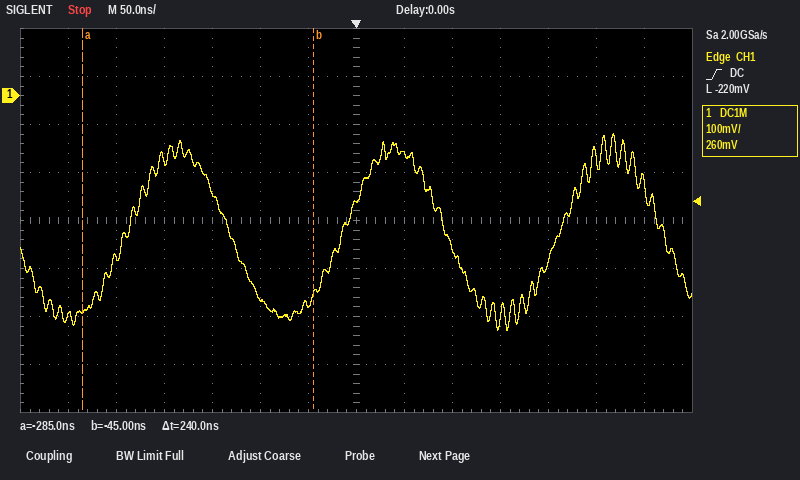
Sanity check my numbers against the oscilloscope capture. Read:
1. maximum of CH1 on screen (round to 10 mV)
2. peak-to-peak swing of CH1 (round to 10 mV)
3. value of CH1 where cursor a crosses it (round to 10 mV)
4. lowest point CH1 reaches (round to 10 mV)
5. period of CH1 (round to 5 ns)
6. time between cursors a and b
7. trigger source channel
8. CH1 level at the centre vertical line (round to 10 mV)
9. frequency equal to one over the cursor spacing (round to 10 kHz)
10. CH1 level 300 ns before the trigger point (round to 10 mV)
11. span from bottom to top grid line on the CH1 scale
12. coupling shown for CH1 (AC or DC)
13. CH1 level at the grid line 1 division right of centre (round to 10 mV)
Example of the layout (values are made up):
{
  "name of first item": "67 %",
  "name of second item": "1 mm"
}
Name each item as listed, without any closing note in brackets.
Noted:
{
  "maximum of CH1 on screen": "-80 mV",
  "peak-to-peak swing of CH1": "410 mV",
  "value of CH1 where cursor a crosses it": "-450 mV",
  "lowest point CH1 reaches": "-490 mV",
  "period of CH1": "225 ns",
  "time between cursors a and b": "240 ns",
  "trigger source channel": "CH1",
  "CH1 level at the centre vertical line": "-220 mV",
  "frequency equal to one over the cursor spacing": "4.17 MHz",
  "CH1 level 300 ns before the trigger point": "-460 mV",
  "span from bottom to top grid line on the CH1 scale": "800 mV",
  "coupling shown for CH1": "DC",
  "CH1 level at the grid line 1 division right of centre": "-120 mV"
}
